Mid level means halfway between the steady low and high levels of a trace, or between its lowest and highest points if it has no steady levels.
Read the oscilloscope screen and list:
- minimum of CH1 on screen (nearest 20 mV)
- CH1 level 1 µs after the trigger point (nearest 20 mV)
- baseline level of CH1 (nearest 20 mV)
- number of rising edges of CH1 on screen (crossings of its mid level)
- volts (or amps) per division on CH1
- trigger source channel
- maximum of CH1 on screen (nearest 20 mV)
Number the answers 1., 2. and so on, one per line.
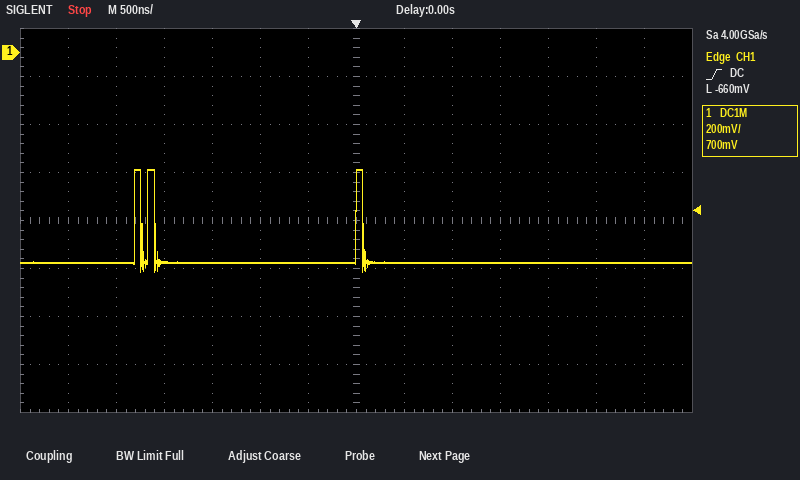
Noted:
1. -920 mV
2. -880 mV
3. -880 mV
4. 3
5. 200 mV
6. CH1
7. -480 mV
